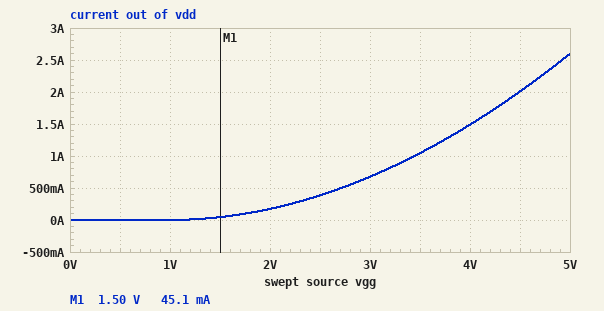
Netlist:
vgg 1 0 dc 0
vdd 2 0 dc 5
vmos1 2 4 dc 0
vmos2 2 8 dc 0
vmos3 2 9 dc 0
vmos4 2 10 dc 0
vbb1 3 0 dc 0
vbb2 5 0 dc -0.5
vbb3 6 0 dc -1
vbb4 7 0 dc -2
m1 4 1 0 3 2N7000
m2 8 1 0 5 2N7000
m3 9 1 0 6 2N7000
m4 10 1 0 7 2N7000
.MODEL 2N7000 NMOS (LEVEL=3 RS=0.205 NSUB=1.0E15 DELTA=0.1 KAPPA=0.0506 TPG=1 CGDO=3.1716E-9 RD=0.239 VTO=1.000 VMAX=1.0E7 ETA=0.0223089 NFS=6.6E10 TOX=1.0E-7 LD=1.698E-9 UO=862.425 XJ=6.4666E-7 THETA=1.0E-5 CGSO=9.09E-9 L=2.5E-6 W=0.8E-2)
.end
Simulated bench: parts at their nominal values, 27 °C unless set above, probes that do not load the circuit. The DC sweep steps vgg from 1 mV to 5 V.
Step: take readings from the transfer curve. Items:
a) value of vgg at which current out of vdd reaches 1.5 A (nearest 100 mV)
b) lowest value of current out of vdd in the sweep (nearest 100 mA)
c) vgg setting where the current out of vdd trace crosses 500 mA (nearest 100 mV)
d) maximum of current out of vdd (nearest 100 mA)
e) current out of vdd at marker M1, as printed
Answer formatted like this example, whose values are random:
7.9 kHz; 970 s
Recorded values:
4.0 V; 0 A; 2.7 V; 2.6 A; 45.1 mA
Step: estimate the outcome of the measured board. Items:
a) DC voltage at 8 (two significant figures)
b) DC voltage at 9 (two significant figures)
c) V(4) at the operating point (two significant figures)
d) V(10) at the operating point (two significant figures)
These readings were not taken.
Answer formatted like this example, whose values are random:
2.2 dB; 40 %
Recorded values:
5.0 V; 5.0 V; 5.0 V; 5.0 V
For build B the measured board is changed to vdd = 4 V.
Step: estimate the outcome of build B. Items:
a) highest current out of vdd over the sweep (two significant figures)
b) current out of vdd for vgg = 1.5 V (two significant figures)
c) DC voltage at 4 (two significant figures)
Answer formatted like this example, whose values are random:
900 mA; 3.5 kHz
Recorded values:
2.6 A; 44 mA; 4.0 V
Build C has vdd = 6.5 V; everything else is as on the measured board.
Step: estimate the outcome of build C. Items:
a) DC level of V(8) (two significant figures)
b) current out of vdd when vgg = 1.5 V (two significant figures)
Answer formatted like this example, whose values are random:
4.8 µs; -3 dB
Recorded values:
6.5 V; 46 mA
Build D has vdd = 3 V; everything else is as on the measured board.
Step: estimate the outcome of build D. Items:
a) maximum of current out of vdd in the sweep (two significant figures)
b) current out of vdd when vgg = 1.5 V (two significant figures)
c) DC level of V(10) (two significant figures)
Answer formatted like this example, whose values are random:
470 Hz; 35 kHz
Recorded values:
2.5 A; 44 mA; 3.0 V
